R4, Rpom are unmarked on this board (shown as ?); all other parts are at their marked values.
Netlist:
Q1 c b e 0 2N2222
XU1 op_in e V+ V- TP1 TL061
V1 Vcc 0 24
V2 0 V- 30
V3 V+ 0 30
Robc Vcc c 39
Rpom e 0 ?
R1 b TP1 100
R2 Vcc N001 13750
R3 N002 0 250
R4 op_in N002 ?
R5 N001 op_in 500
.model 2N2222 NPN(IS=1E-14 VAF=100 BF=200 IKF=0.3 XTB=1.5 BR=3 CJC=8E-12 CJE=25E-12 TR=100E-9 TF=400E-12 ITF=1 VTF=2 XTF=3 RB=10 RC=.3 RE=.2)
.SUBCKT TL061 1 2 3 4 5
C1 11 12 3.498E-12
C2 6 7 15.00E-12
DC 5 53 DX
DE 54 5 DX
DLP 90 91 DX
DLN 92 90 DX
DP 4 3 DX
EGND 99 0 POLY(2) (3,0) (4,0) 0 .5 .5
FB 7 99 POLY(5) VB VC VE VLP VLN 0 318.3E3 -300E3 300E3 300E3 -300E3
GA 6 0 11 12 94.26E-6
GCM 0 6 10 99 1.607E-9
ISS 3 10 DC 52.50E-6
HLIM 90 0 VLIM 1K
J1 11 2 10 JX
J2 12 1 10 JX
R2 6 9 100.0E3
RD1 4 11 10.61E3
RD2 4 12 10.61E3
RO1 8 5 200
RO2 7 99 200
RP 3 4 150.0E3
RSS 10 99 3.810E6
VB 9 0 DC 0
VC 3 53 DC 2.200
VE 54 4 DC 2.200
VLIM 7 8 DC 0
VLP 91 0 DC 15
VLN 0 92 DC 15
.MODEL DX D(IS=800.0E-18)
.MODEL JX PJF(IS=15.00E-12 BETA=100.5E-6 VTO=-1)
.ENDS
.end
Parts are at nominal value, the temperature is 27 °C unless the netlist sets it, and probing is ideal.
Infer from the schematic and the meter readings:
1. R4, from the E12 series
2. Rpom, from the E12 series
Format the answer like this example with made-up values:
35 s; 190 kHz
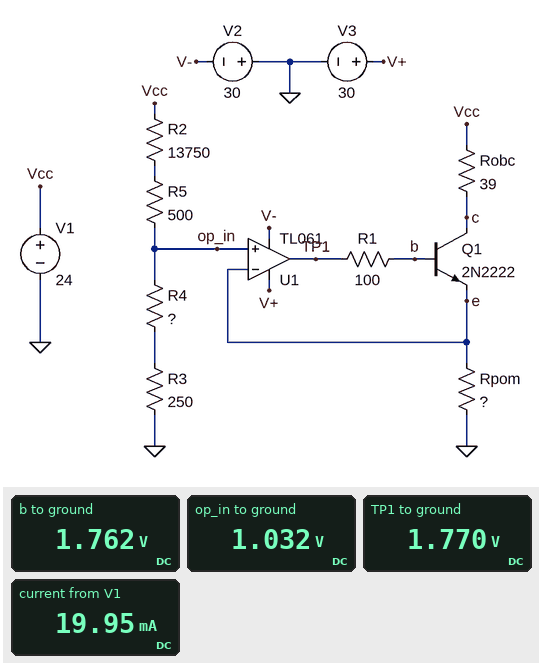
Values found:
390 Ω; 56 Ω
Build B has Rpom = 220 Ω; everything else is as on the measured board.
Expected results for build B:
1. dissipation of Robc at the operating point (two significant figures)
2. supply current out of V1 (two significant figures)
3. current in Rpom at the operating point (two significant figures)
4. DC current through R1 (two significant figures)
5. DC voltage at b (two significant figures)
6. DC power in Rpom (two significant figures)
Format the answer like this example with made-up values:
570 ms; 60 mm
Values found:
850 µW; 6.3 mA; 4.7 mA; 19 µA; 1.7 V; 4.8 mW
